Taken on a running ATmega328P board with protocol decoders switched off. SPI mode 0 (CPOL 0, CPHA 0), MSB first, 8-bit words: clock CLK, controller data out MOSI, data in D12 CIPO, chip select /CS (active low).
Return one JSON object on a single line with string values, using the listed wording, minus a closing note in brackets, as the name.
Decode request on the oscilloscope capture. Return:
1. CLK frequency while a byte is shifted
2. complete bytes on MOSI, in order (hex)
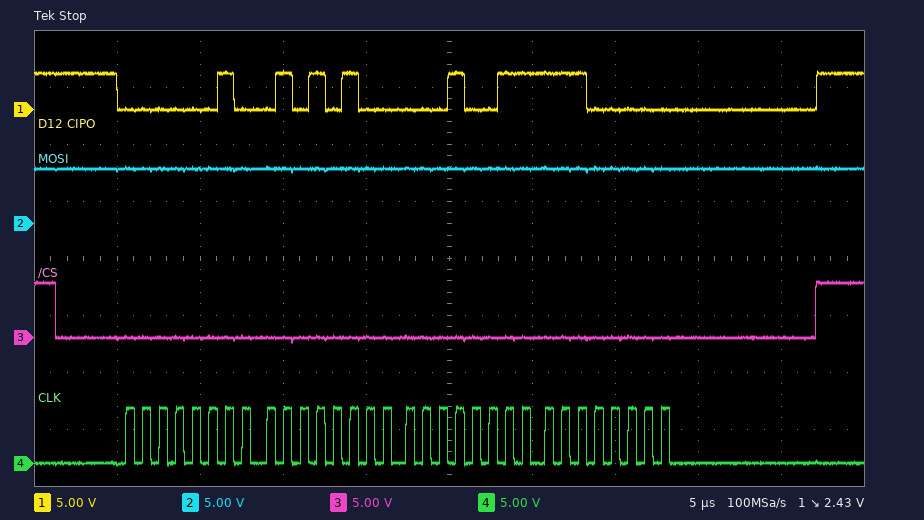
{"CLK frequency while a byte is shifted": "1 MHz", "complete bytes on MOSI, in order": "FF FF FF FF"}
